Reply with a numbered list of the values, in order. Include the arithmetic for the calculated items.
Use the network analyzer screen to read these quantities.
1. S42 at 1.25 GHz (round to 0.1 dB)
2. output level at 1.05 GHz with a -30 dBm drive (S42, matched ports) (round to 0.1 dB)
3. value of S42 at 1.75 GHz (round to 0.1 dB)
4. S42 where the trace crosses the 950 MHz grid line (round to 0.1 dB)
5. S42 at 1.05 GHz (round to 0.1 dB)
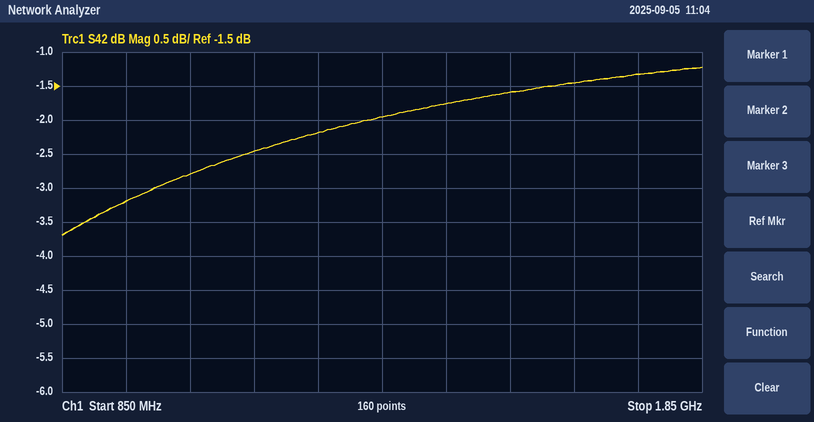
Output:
1. -2.2 dB
2. -30 dBm + (-2.8 dB) = -32.8 dBm
3. -1.3 dB
4. -3.2 dB
5. -2.8 dB
